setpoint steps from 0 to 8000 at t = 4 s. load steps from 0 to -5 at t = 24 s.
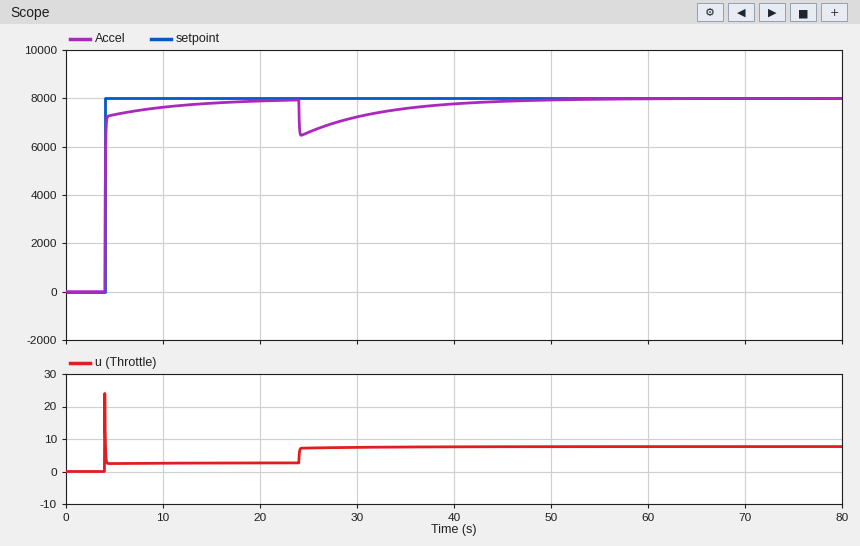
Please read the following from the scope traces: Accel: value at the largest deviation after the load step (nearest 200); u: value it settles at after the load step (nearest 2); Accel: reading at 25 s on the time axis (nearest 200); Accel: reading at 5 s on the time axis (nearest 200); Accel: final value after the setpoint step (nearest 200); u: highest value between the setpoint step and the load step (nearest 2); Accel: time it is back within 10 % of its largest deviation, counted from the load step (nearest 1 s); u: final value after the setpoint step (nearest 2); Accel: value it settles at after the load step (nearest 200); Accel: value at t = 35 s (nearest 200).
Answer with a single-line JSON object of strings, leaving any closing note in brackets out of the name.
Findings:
{"Accel: value at the largest deviation after the load step": "6400", "u: value it settles at after the load step": "8", "Accel: reading at 25 s on the time axis": "6600", "Accel: reading at 5 s on the time axis": "7400", "Accel: final value after the setpoint step": "8000", "u: highest value between the setpoint step and the load step": "24", "Accel: time it is back within 10 % of its largest deviation, counted from the load step": "20 s", "u: final value after the setpoint step": "2", "Accel: value it settles at after the load step": "8000", "Accel: value at t = 35 s": "7600"}
